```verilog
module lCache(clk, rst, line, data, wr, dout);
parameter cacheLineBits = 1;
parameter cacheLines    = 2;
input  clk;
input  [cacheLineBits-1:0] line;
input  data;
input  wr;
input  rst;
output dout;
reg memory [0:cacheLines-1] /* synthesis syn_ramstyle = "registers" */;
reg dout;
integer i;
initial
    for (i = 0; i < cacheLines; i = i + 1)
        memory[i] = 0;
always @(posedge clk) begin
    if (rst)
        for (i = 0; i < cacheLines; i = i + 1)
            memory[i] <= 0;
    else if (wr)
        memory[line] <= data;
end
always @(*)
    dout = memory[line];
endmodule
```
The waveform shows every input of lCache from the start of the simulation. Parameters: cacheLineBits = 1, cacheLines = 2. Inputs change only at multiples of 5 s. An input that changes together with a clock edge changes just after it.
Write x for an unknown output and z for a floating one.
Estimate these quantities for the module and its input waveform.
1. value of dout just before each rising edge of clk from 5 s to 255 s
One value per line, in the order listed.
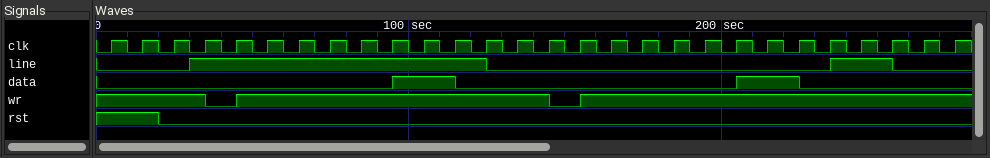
0 0 0 0 0 0 0 0 0 0 0 1 1 0 0 0 0 0 0 0 0 0 1 1 0 0
